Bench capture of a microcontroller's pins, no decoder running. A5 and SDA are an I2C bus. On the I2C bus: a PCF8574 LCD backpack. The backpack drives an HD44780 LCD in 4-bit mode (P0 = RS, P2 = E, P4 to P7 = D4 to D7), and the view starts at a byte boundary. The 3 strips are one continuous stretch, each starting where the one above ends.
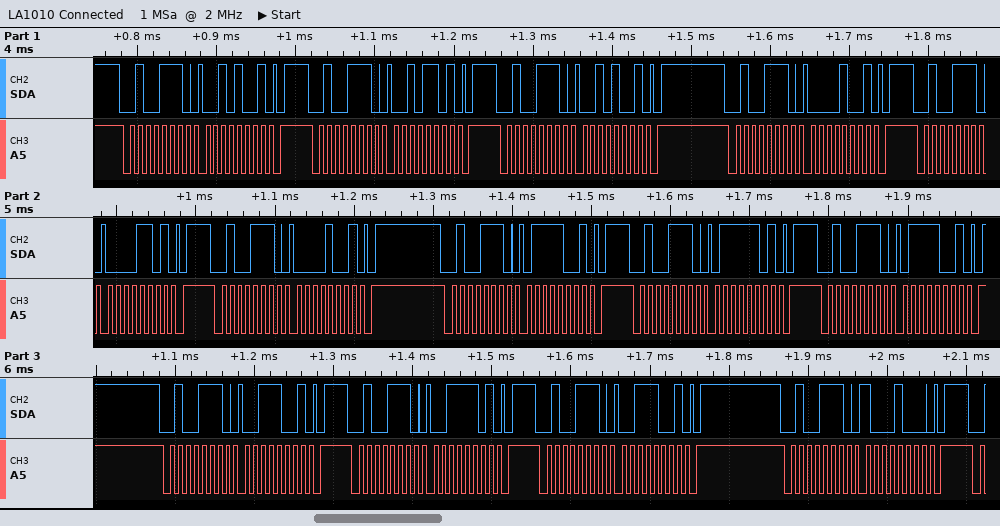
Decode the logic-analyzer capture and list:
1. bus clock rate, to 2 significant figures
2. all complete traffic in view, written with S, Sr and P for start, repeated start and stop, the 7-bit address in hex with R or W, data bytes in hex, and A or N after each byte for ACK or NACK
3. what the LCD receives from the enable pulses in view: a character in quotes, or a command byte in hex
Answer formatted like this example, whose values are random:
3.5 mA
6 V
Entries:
100 kHz
S 27W A 29 A P S 27W A 2D A P S 27W A 29 A P S 27W A 09 A P S 27W A 0D A P S 27W A 09 A P S 27W A 79 A P S 27W A 7D A P S 27W A 79 A P S 27W A 39 A P S 27W A 3D A P S 27W A 39 A P S 27W A 88 A P
' ' 's'
